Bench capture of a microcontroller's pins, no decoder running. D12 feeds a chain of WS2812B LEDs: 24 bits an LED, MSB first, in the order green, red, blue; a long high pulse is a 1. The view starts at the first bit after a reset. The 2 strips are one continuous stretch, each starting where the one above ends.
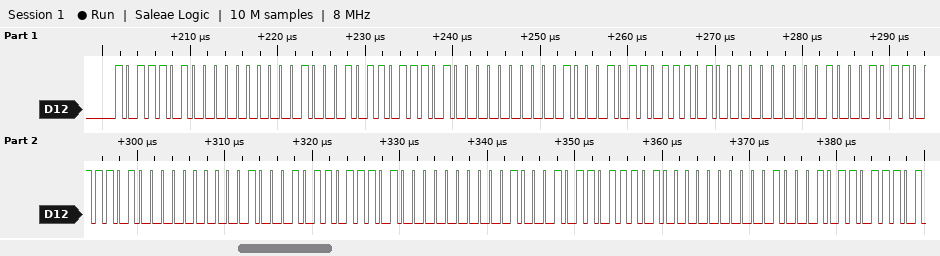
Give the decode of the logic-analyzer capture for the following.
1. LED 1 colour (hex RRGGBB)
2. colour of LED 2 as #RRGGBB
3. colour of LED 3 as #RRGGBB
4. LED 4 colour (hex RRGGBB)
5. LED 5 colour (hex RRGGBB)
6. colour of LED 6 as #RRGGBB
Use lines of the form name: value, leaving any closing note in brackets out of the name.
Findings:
LED 1 colour: #00BA45
colour of LED 2 as #RRGGBB: #00BA45
colour of LED 3 as #RRGGBB: #00BA45
LED 4 colour: #00BA45
LED 5 colour: #00BA45
colour of LED 6 as #RRGGBB: #00BA45
